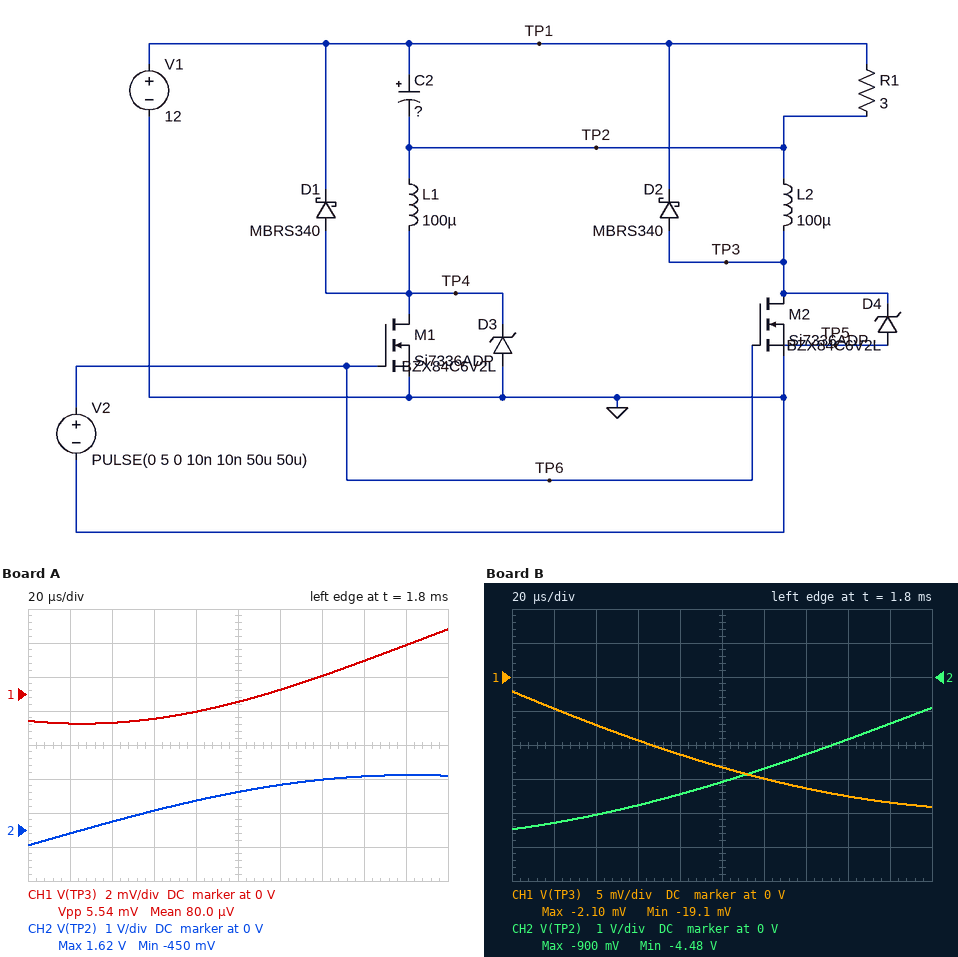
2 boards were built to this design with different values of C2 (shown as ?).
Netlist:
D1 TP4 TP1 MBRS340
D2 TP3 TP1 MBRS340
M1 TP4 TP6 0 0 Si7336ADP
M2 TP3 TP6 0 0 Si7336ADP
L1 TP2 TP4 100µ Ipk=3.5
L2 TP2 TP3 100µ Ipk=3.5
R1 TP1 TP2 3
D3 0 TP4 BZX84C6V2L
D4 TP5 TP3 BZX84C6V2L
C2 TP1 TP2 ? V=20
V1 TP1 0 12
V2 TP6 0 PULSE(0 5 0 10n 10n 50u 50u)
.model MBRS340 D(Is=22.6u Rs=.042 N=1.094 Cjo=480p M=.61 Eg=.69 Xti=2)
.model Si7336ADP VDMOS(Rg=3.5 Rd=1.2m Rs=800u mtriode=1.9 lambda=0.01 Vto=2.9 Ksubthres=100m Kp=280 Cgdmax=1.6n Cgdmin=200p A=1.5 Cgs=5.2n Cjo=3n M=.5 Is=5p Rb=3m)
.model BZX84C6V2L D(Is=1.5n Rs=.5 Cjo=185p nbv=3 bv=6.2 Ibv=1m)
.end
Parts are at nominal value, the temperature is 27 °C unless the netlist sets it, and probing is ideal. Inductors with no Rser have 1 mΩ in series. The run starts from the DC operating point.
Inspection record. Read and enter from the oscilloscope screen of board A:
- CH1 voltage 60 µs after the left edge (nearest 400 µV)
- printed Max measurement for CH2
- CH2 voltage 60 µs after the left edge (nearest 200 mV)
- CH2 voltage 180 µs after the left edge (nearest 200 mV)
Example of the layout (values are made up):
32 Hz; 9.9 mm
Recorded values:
-1.6 mV; 1.62 V; 600 mV; 1.6 V
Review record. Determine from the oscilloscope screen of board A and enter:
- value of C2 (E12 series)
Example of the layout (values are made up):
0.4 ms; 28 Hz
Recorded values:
220 µF
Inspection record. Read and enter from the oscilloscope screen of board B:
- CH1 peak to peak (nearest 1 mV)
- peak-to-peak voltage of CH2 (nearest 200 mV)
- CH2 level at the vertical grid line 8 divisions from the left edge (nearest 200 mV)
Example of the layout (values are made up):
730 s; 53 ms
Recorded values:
17 mV; 3.6 V; -1.8 V
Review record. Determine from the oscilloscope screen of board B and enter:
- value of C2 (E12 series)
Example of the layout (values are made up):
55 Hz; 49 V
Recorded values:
680 µF
